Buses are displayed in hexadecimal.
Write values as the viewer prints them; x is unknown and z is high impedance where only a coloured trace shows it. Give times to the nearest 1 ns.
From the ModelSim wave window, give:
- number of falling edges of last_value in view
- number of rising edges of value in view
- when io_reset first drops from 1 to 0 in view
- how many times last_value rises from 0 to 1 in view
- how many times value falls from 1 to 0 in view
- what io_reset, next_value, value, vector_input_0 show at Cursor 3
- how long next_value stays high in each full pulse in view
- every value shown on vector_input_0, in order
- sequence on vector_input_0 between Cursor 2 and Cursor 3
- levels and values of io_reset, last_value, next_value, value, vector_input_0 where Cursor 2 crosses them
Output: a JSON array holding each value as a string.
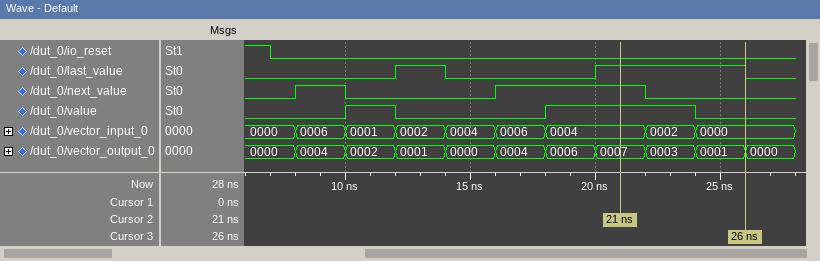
["2", "2", "7 ns", "2", "2", "io_reset=0, next_value=0, value=0, vector_input_0=0000", "2 ns, 6 ns", "0000, 0006, 0001, 0002, 0004, 0006, 0004, 0002, 0000", "0004, 0002, 0000", "io_reset=0, last_value=1, next_value=1, value=1, vector_input_0=0004"]
